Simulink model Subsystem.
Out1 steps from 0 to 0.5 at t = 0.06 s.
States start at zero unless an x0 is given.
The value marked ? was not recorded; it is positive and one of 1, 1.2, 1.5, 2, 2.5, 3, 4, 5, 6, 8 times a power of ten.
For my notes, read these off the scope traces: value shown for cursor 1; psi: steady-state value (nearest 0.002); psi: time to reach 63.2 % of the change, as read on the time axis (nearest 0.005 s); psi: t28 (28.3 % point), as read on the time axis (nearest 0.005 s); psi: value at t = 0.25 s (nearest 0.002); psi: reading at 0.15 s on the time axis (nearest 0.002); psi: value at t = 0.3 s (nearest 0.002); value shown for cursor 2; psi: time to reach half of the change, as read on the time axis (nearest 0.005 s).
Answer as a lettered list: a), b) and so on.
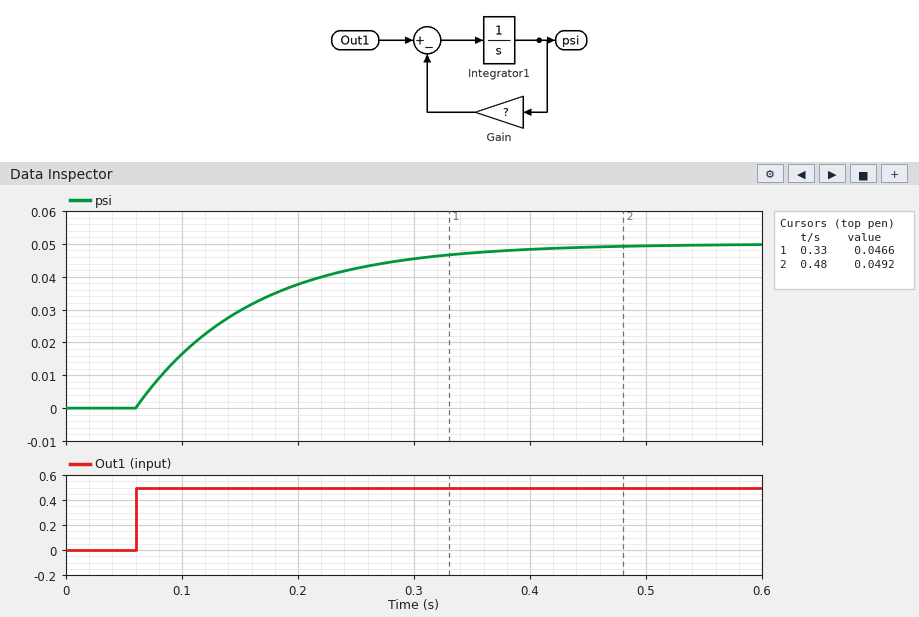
a) 0.0466
b) 0.050
c) 0.160 s
d) 0.095 s
e) 0.042
f) 0.030
g) 0.046
h) 0.0492
i) 0.130 s
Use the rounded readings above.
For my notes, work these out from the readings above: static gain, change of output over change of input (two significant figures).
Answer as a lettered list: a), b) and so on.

a) 0.10
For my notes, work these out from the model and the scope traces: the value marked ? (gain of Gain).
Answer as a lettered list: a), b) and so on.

a) 10
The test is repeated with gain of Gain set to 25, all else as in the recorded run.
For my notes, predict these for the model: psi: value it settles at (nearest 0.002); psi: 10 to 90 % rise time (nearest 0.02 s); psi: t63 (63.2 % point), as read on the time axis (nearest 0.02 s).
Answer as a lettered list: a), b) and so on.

a) 0.020
b) 0.08 s
c) 0.10 s
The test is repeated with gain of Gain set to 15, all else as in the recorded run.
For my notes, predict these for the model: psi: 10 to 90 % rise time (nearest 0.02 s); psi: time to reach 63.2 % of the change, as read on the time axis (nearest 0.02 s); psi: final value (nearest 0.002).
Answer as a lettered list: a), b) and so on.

a) 0.14 s
b) 0.12 s
c) 0.034
